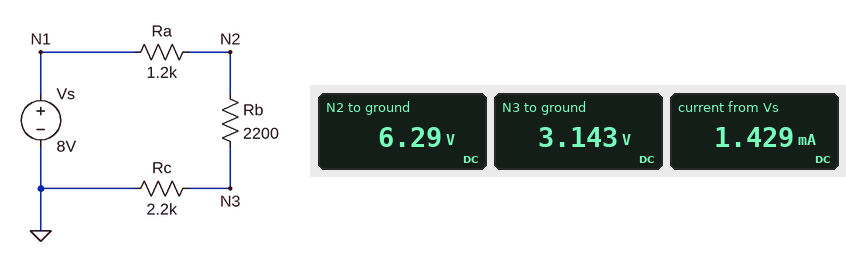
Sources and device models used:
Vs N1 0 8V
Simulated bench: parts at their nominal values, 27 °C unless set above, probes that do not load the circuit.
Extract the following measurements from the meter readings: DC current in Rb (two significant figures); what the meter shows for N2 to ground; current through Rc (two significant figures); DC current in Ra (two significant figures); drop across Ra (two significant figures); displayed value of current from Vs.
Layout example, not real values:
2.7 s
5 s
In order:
1.4 mA
6.29 V
1.4 mA
1.4 mA
1.7 V
1.429 mA
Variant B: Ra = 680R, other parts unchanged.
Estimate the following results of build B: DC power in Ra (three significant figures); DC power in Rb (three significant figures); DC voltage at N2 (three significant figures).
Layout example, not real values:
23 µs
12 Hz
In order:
1.69 mW
5.46 mW
6.93 V
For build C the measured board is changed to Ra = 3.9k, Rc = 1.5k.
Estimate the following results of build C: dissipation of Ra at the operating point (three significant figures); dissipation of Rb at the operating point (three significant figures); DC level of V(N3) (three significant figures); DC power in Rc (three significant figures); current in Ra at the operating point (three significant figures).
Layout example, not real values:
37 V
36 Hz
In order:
4.32 mW
2.44 mW
1.58 V
1.66 mW
1.05 mA
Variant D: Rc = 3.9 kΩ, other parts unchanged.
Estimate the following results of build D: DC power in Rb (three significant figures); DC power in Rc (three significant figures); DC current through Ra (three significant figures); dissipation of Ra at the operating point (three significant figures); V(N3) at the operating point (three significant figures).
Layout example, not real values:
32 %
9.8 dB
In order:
2.64 mW
4.68 mW
1.10 mA
1.44 mW
4.27 V
